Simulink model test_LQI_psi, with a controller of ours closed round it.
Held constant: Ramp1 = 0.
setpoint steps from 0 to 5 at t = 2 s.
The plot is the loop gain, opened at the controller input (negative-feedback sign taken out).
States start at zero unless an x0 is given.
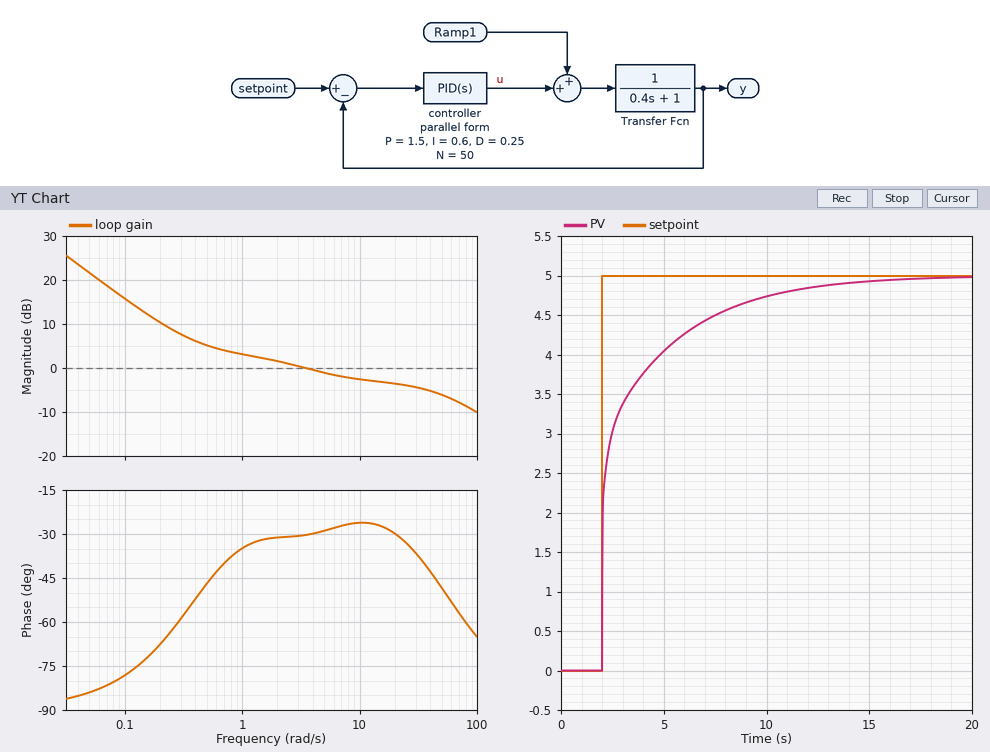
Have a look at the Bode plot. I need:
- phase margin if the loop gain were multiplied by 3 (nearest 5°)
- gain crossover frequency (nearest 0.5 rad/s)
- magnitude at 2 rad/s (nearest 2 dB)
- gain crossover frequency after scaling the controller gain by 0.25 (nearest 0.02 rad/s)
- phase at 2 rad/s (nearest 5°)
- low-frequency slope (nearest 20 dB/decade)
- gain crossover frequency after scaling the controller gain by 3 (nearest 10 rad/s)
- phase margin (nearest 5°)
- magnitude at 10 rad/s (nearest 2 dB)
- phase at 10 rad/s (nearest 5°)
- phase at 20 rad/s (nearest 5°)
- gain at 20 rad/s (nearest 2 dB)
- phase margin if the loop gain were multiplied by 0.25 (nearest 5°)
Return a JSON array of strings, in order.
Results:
["115°", "3.5 rad/s", "2 dB", "0.16 rad/s", "-30°", "-20 dB/decade", "90 rad/s", "150°", "-2 dB", "-25°", "-30°", "-4 dB", "110°"]
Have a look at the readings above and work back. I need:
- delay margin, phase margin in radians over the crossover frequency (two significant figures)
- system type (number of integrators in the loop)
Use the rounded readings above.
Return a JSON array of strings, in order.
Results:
["0.75 s", "1"]
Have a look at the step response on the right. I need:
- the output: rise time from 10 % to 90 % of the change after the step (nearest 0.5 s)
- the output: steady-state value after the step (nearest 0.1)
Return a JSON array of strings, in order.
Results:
["5.5 s", "5.0"]
